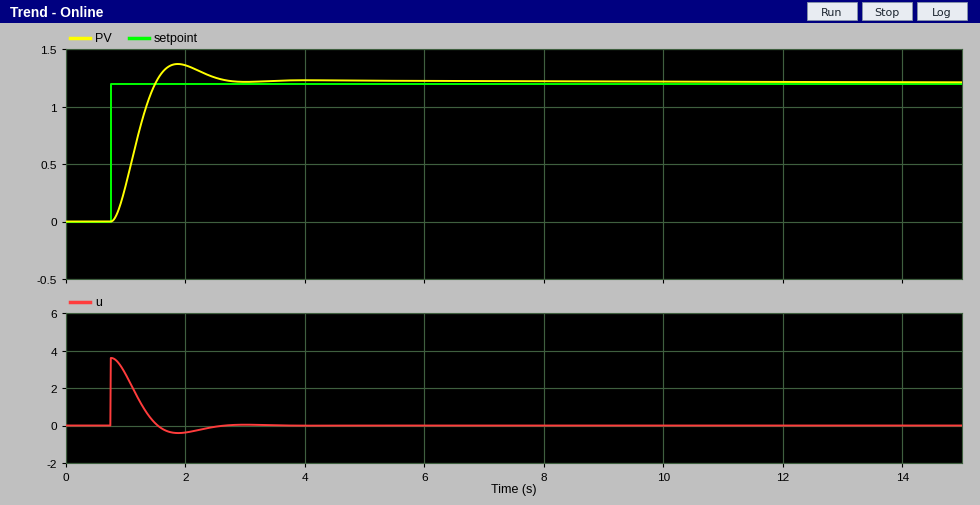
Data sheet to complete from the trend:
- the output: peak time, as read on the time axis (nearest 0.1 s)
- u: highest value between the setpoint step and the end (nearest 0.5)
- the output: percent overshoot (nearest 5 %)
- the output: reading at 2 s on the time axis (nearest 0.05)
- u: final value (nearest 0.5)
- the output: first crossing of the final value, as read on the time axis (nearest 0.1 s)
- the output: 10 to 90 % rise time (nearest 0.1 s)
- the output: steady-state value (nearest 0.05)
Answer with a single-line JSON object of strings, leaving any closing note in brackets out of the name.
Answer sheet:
{"the output: peak time, as read on the time axis": "1.9 s", "u: highest value between the setpoint step and the end": "3.5", "the output: percent overshoot": "15 %", "the output: reading at 2 s on the time axis": "1.35", "u: final value": "0.0", "the output: first crossing of the final value, as read on the time axis": "1.5 s", "the output: 10 to 90 % rise time": "0.5 s", "the output: steady-state value": "1.20"}
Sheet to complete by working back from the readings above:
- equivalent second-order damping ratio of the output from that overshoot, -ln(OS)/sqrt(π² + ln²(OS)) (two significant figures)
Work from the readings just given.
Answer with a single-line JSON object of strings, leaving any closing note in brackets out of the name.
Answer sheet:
{"equivalent second-order damping ratio of the output from that overshoot, -ln(OS)/sqrt(π² + ln²(OS))": "0.52"}
